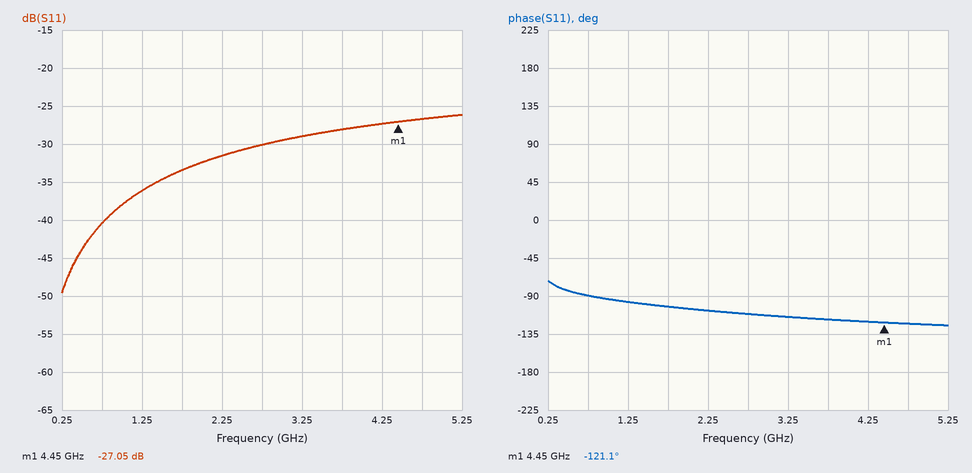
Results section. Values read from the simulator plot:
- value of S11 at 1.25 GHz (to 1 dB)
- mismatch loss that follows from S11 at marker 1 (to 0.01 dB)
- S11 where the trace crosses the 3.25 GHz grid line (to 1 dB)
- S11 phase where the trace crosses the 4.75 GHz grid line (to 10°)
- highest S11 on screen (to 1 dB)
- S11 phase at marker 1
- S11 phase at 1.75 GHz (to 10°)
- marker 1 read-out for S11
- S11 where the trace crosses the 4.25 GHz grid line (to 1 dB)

-36 dB
0.01 dB
-29 dB
-120°
-26 dB
-121.1°
-100°
-27.05 dB
-27 dB
